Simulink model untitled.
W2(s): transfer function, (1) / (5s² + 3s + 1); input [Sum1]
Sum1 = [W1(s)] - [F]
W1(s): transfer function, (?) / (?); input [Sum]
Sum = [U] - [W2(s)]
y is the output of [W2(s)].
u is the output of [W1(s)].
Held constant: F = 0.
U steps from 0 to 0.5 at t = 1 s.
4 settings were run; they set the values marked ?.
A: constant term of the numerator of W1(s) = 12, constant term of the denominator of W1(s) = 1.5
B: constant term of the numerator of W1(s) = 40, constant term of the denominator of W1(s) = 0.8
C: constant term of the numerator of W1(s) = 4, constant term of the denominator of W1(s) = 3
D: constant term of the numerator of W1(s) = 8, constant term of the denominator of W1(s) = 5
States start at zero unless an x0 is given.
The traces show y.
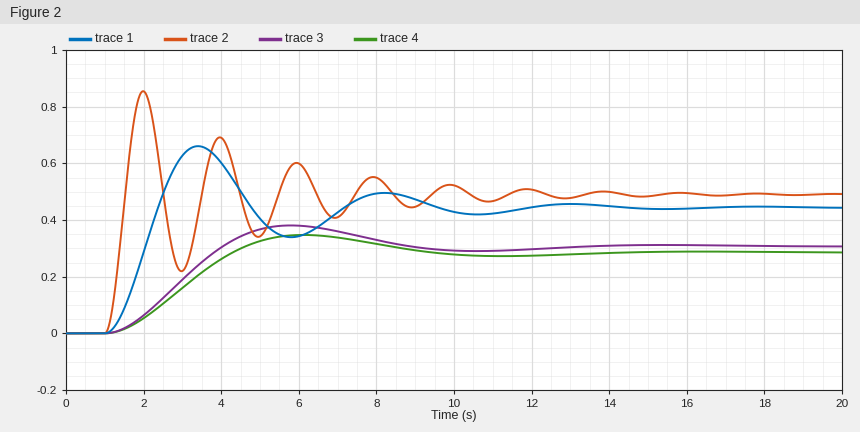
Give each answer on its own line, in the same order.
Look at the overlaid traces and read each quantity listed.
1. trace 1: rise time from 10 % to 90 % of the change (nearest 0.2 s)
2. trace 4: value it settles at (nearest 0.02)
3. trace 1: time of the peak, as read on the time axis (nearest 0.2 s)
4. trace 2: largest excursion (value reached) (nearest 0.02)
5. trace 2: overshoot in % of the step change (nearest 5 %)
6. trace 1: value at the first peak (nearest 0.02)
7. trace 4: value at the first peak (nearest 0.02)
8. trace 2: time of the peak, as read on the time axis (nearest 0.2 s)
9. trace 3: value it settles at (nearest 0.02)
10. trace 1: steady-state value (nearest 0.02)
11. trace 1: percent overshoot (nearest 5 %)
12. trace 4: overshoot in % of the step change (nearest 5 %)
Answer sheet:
1.0 s
0.28
3.4 s
0.86
75 %
0.66
0.34
2.0 s
0.30
0.44
50 %
20 %
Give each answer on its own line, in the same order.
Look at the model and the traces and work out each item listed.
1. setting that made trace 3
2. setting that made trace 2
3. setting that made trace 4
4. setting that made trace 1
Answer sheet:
D
B
C
A
